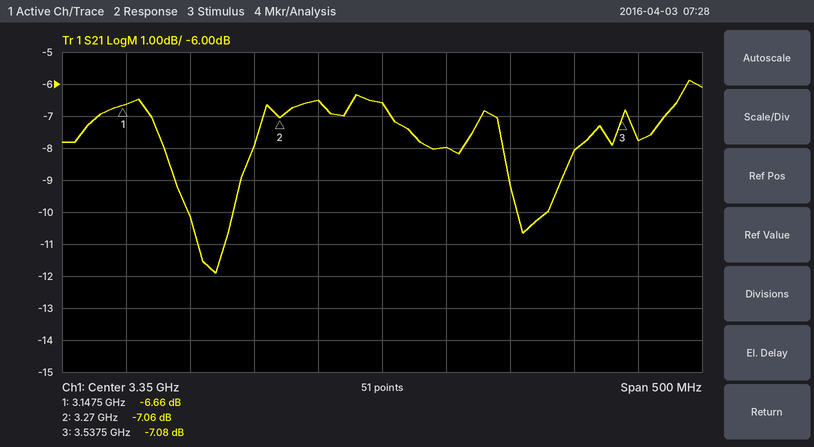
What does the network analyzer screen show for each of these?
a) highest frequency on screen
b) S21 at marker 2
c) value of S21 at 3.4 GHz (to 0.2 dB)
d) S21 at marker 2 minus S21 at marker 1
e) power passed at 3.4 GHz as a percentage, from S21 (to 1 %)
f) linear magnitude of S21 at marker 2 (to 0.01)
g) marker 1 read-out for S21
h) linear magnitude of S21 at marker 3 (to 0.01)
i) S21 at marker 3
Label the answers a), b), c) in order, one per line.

a) 3.6 GHz
b) -7.06 dB
c) -8.0 dB
d) -0.40 dB
e) 16 %
f) 0.44
g) -6.66 dB
h) 0.44
i) -7.08 dB
